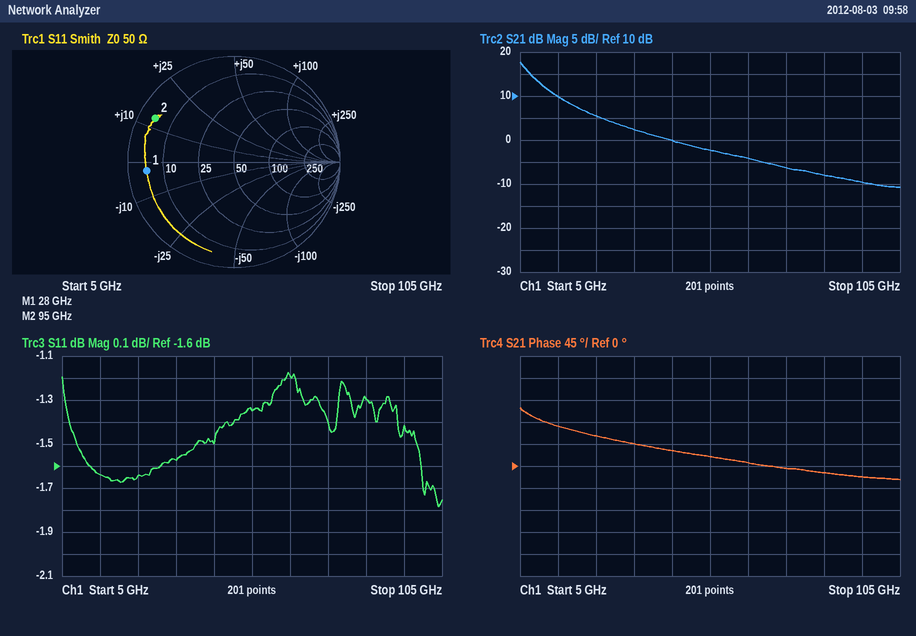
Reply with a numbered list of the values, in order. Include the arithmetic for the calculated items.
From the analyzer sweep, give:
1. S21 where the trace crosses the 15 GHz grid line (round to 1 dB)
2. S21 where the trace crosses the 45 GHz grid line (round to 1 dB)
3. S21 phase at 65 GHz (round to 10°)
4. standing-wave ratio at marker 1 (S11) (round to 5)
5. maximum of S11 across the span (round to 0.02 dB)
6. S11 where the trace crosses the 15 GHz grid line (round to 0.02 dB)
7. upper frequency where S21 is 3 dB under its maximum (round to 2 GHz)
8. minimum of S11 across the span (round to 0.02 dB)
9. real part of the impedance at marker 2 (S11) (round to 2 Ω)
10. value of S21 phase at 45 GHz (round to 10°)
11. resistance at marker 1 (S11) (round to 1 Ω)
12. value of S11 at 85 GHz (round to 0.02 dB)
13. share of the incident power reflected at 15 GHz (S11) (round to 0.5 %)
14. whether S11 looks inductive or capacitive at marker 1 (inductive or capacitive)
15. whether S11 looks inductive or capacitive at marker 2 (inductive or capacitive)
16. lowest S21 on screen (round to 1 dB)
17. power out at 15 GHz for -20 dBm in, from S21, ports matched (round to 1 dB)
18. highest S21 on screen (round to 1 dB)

1. 10 dB
2. 0 dB
3. 10°
4. 10
5. -1.18 dB
6. -1.64 dB
7. 8 GHz
8. -1.78 dB
9. 4 Ω
10. 30°
11. 5 Ω
12. -1.30 dB
13. 10^(-1.64/10) ≈ 68.5 %
14. capacitive
15. inductive
16. -11 dB
17. -20 dBm + (10 dB) = -10 dBm
18. 18 dB
